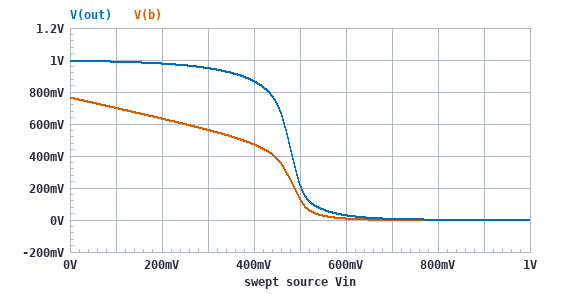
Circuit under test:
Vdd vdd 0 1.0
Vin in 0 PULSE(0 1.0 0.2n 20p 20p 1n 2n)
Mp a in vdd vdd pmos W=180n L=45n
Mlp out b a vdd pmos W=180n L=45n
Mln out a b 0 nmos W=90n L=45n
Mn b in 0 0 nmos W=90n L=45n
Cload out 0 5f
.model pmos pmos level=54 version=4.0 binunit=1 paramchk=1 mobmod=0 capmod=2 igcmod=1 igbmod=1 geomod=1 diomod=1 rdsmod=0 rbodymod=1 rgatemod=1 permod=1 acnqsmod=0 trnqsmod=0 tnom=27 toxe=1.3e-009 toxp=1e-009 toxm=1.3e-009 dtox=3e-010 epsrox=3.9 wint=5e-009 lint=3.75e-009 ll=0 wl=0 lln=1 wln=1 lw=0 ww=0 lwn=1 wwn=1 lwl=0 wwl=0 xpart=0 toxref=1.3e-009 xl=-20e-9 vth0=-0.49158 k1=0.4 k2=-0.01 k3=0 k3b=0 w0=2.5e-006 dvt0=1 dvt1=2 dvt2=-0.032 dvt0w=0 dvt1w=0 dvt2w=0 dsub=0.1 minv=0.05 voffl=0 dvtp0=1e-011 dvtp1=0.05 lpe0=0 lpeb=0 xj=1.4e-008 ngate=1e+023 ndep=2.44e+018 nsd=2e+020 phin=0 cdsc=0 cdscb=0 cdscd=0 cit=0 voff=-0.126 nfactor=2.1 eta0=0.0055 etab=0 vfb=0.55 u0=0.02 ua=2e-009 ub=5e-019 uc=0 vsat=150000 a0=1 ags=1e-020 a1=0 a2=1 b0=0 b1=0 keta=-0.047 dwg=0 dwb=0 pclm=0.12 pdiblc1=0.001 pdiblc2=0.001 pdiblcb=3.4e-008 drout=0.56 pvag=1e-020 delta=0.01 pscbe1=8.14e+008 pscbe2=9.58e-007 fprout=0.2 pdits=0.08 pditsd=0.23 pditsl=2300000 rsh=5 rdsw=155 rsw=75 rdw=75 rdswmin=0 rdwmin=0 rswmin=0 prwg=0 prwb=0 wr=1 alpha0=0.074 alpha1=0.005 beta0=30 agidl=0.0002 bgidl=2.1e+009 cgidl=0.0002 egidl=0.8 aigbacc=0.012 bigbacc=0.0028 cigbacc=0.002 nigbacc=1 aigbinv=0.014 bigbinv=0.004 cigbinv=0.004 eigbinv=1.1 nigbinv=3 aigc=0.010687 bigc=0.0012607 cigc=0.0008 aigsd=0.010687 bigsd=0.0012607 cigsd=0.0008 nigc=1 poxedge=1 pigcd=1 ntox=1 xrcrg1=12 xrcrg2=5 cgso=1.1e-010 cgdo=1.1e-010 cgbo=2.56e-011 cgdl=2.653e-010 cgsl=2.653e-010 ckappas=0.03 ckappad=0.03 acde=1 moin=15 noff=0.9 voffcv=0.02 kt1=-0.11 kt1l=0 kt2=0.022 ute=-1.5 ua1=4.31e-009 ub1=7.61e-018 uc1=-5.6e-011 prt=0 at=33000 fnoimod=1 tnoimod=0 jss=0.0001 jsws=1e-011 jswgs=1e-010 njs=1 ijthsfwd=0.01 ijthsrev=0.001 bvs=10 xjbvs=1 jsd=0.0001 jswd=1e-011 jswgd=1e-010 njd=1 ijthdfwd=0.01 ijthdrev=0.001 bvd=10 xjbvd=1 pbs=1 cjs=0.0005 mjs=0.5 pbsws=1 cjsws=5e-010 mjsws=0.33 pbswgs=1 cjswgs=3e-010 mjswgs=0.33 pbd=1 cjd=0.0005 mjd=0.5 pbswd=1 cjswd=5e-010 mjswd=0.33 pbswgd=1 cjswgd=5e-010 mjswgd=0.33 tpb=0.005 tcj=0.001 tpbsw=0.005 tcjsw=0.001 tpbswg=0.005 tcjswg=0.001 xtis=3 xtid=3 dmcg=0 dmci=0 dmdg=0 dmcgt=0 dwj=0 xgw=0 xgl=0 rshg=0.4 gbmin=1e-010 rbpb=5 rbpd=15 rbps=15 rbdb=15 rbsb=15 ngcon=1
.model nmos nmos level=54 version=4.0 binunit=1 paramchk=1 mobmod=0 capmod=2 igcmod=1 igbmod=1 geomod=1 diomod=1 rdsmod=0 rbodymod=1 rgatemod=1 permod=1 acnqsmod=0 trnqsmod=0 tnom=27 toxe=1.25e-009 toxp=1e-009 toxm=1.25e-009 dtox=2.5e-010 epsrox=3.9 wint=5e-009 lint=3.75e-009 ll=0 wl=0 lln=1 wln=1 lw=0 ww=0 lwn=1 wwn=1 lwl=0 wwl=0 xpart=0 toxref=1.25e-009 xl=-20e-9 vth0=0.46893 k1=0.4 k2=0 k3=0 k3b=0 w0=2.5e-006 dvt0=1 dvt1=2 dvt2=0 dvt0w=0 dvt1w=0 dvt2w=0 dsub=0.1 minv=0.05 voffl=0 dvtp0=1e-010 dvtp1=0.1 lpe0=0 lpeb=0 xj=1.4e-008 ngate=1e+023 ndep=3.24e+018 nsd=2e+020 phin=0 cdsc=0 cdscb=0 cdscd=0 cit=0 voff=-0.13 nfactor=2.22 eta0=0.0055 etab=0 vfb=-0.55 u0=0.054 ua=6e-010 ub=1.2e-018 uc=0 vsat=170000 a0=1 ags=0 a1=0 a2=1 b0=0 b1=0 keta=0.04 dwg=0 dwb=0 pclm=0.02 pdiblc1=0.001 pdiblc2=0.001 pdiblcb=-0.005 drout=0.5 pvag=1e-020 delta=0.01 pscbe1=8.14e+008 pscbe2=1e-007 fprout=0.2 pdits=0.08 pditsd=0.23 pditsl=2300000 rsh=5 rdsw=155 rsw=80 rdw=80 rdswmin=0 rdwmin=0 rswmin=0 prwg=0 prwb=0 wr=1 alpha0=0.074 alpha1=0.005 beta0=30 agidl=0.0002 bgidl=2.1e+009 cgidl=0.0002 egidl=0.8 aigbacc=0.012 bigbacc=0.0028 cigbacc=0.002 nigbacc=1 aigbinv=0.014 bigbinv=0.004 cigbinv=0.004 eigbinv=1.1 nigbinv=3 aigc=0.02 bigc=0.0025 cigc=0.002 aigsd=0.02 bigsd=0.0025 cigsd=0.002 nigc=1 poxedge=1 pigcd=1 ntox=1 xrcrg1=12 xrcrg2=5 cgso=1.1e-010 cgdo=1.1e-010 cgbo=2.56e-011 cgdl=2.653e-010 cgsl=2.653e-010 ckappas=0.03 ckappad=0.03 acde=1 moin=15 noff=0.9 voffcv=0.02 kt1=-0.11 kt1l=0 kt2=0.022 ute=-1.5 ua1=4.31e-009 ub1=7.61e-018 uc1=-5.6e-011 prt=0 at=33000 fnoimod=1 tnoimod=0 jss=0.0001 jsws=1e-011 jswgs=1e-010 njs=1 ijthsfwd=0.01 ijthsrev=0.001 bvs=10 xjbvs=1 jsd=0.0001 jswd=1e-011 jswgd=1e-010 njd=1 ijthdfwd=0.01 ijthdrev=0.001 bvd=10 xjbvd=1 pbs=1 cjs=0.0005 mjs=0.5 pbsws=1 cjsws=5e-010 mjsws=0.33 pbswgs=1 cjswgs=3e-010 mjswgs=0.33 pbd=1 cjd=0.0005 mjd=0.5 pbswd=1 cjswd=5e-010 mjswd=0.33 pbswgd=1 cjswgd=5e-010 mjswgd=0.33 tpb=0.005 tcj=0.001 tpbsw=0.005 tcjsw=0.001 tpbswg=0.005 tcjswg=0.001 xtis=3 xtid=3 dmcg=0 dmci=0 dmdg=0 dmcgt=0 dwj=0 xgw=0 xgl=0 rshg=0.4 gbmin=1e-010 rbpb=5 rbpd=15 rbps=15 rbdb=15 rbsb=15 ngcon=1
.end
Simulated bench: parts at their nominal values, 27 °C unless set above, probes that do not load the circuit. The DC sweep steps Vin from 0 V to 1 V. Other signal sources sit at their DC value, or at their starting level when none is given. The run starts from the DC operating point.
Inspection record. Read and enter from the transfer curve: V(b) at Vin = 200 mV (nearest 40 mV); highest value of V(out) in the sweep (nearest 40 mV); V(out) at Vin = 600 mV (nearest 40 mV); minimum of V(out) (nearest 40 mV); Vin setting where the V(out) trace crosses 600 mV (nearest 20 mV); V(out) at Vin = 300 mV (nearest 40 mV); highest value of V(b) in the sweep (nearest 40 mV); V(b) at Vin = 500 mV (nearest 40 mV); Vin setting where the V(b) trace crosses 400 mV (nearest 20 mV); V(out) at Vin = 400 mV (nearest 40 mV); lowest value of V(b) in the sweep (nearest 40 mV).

640 mV
1.00 V
40 mV
0 V
460 mV
960 mV
760 mV
120 mV
440 mV
880 mV
0 V
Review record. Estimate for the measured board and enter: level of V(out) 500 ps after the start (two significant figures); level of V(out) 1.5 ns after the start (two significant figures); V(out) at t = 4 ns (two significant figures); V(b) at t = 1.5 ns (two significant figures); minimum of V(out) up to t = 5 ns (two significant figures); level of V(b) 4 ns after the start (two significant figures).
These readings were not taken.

280 mV
620 mV
680 mV
590 mV
120 mV
640 mV
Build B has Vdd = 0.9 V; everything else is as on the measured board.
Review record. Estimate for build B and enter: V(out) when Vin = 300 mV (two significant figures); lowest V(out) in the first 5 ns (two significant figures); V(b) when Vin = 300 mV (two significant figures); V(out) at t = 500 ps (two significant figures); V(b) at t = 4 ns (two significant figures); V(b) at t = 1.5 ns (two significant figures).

830 mV
150 mV
480 mV
300 mV
550 mV
490 mV
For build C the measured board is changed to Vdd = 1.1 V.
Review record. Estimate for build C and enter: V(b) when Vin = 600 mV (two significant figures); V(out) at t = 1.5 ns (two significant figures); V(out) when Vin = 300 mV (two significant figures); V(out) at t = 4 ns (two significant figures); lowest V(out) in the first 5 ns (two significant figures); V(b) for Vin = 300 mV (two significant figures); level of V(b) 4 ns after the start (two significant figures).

53 mV
720 mV
1.1 V
790 mV
83 mV
640 mV
740 mV
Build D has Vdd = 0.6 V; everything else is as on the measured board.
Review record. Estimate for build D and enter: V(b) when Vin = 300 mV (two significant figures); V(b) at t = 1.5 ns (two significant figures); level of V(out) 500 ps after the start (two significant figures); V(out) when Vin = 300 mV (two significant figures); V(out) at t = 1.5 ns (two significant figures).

25 mV
250 mV
330 mV
36 mV
260 mV
